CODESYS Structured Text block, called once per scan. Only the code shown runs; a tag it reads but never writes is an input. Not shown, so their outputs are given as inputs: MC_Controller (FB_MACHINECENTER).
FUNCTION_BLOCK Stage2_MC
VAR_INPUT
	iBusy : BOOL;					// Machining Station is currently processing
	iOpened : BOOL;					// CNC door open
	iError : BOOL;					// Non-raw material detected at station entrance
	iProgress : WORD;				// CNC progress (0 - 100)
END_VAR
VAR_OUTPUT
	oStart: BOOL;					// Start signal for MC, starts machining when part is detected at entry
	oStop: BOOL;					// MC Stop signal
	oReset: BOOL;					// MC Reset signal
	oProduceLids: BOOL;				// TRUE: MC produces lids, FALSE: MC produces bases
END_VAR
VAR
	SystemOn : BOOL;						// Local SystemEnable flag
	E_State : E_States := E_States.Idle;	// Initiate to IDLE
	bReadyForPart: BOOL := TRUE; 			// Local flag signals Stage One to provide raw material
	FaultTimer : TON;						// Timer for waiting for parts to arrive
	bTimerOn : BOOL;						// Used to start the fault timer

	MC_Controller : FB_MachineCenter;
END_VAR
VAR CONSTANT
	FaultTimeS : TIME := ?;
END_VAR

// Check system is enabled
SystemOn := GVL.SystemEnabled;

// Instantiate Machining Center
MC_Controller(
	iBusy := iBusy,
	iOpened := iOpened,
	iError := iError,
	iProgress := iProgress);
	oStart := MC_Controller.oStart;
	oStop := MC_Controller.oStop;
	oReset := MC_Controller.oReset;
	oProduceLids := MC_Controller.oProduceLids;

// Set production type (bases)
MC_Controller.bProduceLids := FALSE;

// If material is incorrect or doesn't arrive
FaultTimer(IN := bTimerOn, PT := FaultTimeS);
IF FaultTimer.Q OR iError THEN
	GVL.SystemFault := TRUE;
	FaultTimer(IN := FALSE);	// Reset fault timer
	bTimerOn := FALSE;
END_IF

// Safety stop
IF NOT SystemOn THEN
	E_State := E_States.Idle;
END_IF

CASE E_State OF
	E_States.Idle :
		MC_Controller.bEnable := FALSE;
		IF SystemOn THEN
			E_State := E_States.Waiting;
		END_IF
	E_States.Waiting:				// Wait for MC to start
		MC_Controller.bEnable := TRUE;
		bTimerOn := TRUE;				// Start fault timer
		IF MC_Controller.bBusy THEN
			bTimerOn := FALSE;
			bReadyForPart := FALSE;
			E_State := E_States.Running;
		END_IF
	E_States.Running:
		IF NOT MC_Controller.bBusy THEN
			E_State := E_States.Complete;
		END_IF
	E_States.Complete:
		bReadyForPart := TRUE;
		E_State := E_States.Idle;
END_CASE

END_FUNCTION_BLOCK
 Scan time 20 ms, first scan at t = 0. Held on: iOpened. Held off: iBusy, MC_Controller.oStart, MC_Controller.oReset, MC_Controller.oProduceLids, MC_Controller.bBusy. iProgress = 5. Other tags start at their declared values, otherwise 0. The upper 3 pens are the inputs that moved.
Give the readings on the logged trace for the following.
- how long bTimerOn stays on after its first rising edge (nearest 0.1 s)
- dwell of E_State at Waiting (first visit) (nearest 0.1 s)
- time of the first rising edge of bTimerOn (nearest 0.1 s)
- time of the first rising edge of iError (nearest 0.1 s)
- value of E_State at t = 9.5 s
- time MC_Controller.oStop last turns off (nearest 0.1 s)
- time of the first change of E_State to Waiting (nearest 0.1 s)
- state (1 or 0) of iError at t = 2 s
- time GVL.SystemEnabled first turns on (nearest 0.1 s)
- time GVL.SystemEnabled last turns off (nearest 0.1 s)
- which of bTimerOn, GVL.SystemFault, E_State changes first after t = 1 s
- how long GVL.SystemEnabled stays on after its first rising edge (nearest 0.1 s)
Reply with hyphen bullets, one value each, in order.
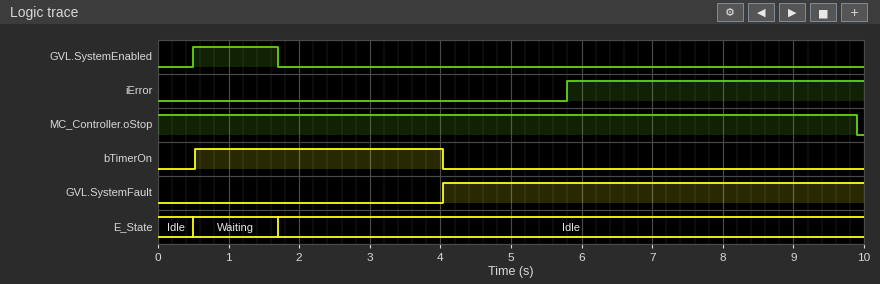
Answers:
- 3.5 s
- 1.2 s
- 0.5 s
- 5.8 s
- Idle
- 9.9 s
- 0.5 s
- 0
- 0.5 s
- 1.7 s
- E_State
- 1.2 s
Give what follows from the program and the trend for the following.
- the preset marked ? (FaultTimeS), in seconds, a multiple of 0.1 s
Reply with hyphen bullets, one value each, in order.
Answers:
- 3.5 s
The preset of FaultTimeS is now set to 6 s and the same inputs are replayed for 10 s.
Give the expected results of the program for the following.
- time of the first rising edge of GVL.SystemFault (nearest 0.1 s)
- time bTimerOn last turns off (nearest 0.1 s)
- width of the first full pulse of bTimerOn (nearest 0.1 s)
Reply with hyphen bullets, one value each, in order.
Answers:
- 5.8 s
- 5.8 s
- 5.3 s
